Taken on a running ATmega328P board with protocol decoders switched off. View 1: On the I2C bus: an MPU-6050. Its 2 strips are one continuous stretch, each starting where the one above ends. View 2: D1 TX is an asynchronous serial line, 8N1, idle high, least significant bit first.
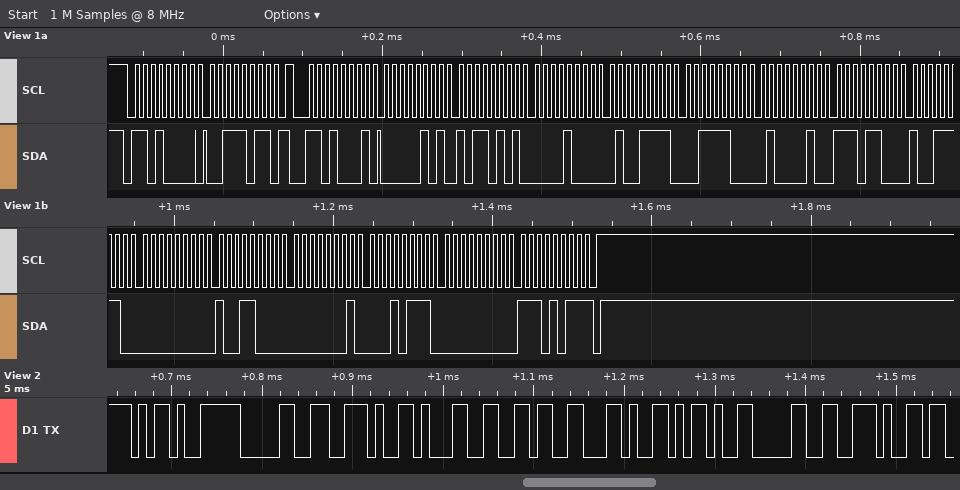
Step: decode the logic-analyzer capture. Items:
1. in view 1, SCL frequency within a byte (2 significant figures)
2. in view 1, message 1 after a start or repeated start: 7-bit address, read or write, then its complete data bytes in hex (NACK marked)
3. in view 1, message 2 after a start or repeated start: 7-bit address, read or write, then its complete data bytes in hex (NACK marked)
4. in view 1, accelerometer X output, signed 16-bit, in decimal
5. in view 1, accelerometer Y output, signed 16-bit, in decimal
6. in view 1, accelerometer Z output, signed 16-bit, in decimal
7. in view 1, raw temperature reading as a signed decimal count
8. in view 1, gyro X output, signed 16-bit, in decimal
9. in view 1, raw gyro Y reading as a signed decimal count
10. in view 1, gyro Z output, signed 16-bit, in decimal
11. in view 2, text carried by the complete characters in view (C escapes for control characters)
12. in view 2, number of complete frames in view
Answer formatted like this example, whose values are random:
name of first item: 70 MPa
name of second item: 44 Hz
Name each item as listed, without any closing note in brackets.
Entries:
in view 1, SCL frequency within a byte: 100 kHz
in view 1, message 1 after a start or repeated start: 7-bit address, read or write, then its complete data bytes in hex: 0x68 write: 3B
in view 1, message 2 after a start or repeated start: 7-bit address, read or write, then its complete data bytes in hex: 0x68 read: 05 B5 08 4F 3C 42 EC 9E 00 98 01 17 00 EB NACK
in view 1, accelerometer X output, signed 16-bit, in decimal: 1461
in view 1, accelerometer Y output, signed 16-bit, in decimal: 2127
in view 1, accelerometer Z output, signed 16-bit, in decimal: 15426
in view 1, raw temperature reading as a signed decimal count: -4962
in view 1, gyro X output, signed 16-bit, in decimal: 152
in view 1, raw gyro Y reading as a signed decimal count: 279
in view 1, gyro Z output, signed 16-bit, in decimal: 235
in view 2, text carried by the complete characters in view: "-0.16,-0."
in view 2, number of complete frames in view: 9
